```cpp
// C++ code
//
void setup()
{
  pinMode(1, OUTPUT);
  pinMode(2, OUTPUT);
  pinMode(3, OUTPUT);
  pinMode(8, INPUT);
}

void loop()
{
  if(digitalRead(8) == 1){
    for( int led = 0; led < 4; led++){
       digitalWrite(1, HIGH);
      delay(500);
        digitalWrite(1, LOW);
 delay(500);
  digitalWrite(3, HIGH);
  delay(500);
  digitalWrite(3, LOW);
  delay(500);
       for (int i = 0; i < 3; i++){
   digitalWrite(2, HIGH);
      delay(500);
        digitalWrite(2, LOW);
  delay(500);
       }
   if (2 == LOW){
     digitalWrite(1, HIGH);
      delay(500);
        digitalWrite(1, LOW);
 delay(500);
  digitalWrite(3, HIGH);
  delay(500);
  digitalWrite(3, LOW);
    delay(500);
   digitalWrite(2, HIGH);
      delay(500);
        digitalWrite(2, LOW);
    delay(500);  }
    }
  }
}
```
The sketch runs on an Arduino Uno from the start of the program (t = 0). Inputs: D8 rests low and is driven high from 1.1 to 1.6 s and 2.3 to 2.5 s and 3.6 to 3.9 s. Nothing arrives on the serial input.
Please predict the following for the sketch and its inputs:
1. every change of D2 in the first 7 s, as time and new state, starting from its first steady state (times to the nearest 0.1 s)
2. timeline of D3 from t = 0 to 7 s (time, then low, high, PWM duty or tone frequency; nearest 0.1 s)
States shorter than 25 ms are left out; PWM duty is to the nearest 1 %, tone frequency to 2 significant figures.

0 s low; 3.1 s high; 3.6 s low; 4.1 s high; 4.6 s low; 5.1 s high; 5.6 s low
0 s low; 2.1 s high; 2.6 s low
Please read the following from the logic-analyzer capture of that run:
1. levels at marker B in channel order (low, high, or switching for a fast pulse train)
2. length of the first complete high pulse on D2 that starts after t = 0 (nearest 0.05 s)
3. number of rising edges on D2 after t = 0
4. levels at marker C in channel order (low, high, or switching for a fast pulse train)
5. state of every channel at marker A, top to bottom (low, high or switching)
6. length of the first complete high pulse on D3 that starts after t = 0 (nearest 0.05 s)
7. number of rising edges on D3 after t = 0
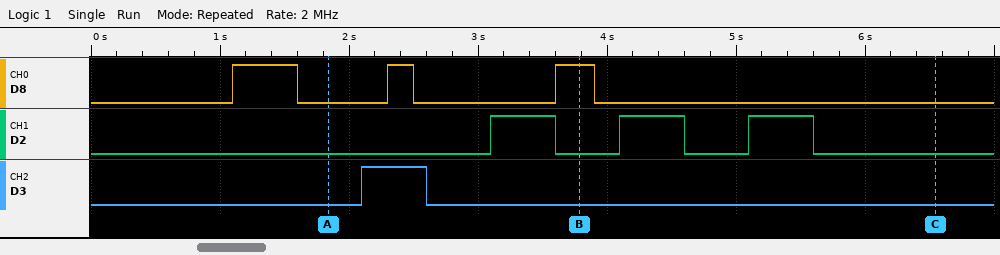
D8 high, D2 low, D3 low
0.50 s
3
D8 low, D2 low, D3 low
D8 low, D2 low, D3 low
0.50 s
1
